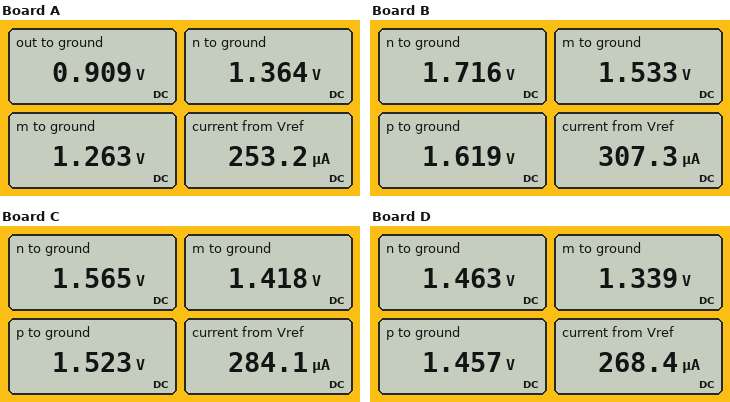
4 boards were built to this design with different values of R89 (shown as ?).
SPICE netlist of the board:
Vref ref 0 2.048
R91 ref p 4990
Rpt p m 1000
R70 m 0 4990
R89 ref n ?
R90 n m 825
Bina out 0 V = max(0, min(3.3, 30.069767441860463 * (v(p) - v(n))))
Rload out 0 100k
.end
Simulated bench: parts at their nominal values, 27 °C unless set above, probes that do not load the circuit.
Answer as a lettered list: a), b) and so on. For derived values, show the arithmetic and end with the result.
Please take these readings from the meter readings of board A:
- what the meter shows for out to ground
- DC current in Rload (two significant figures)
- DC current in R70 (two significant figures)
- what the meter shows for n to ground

a) 0.909 V
b) (909 mV) / 100 kΩ = 9.1 µA
c) (1.263 V) / 4.99 kΩ = 250 µA
d) 1.364 V
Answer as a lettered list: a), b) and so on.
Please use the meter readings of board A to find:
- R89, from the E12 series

a) 5.6 kΩ
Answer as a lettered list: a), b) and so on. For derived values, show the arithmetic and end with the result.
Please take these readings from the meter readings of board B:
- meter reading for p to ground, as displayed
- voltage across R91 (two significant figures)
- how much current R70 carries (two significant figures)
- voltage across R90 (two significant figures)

a) 1.619 V
b) 2.048 V - 1.619 V = 430 mV
c) (1.533 V) / 4.99 kΩ = 310 µA
d) 1.716 V - 1.533 V = 180 mV
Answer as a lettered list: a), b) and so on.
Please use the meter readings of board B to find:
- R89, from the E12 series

a) 1.5 kΩ
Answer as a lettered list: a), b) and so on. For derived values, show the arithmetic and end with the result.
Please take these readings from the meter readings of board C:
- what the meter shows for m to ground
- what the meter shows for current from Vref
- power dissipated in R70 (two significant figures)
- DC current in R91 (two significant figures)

a) 1.418 V
b) 284.1 µA
c) (1.418 V)^2 / 4.99 kΩ = 400 µW
d) (2.048 V - 1.523 V) / 4.99 kΩ = 110 µA
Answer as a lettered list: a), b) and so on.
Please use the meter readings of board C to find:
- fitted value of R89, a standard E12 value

a) 2.7 kΩ
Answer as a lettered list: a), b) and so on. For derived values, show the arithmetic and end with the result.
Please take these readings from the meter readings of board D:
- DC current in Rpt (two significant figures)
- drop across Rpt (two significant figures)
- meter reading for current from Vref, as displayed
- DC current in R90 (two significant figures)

a) (1.457 V - 1.339 V) / 1 kΩ = 120 µA
b) 1.457 V - 1.339 V = 120 mV
c) 268.4 µA
d) (1.463 V - 1.339 V) / 825 Ω = 150 µA
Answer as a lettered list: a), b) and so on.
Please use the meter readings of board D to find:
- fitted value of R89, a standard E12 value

a) 3.9 kΩ
